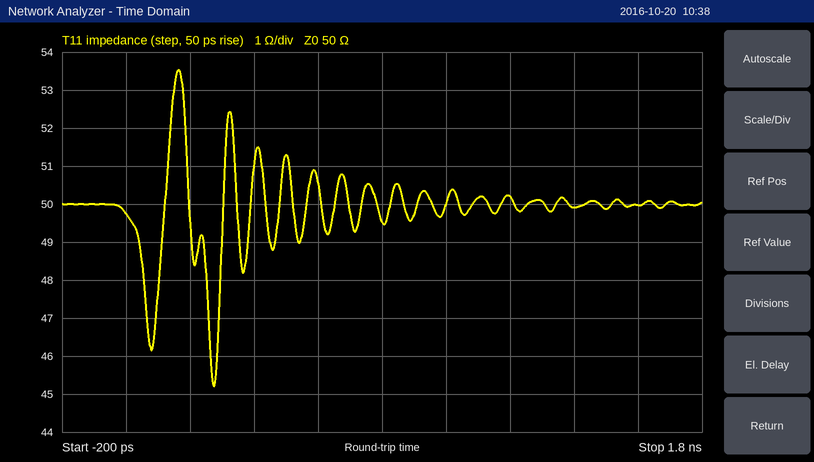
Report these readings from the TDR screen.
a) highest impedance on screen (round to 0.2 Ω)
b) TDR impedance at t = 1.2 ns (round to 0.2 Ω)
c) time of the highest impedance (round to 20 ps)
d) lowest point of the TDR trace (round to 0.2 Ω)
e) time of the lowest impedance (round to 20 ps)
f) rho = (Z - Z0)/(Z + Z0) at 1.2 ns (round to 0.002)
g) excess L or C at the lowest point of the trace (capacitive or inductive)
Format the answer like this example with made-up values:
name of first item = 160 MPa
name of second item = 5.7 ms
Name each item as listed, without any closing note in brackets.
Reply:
highest impedance on screen = 53.6 Ω
TDR impedance at t = 1.2 ns = 50.2 Ω
time of the highest impedance = 160 ps
lowest point of the TDR trace = 45.2 Ω
time of the lowest impedance = 280 ps
rho = (Z - Z0)/(Z + Z0) at 1.2 ns = +0.002
excess L or C at the lowest point of the trace = capacitive
